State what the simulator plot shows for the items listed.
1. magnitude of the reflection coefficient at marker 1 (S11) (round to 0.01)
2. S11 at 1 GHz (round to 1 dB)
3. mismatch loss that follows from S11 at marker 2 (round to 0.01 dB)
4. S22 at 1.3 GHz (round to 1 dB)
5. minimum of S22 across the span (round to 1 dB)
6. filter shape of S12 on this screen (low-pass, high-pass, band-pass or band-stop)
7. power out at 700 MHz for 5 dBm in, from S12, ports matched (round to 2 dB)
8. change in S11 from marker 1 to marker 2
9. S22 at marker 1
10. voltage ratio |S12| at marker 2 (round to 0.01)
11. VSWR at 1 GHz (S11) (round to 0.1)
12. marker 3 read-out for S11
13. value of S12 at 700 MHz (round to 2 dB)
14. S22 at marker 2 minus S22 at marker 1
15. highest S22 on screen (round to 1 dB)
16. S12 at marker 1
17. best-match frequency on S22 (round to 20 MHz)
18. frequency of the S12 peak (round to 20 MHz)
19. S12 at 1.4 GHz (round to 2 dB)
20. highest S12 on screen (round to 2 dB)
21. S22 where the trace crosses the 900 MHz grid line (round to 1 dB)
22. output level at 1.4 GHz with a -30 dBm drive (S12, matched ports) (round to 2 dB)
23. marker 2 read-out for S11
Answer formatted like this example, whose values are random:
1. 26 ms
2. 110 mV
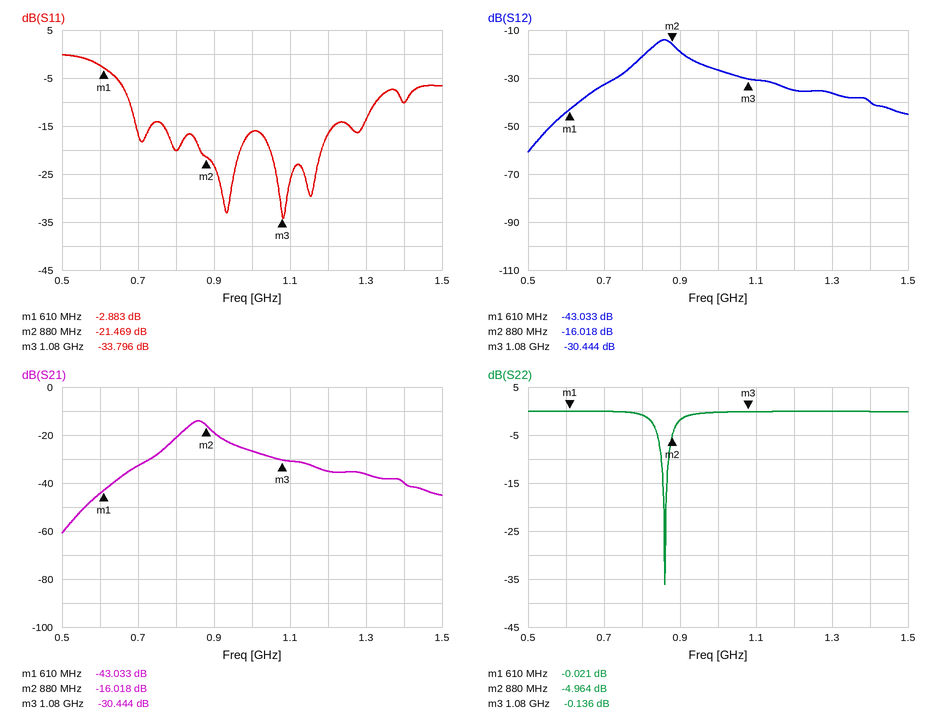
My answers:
1. 0.72
2. -16 dB
3. 0.03 dB
4. 0 dB
5. -36 dB
6. band-pass
7. -28 dBm
8. -18.586 dB
9. -0.021 dB
10. 0.16
11. 1.4
12. -33.796 dB
13. -32 dB
14. -4.943 dB
15. 0 dB
16. -43.033 dB
17. 860 MHz
18. 860 MHz
19. -40 dB
20. -14 dB
21. -2 dB
22. -70 dBm
23. -21.469 dB
